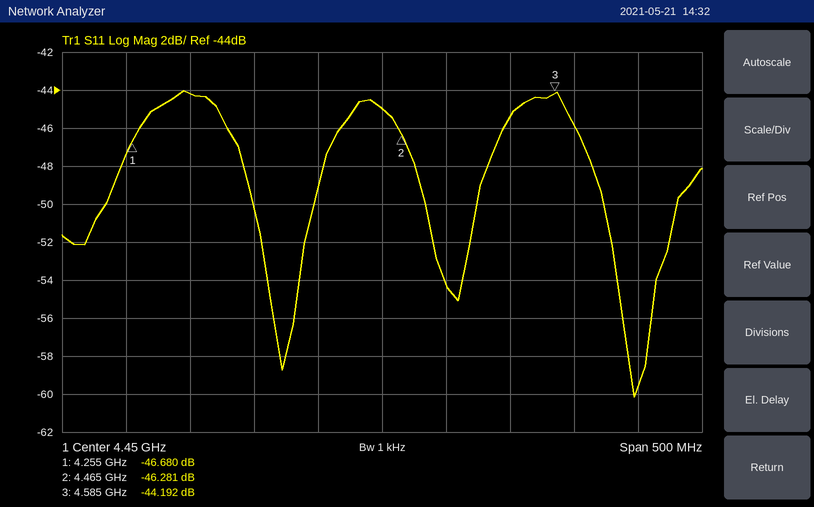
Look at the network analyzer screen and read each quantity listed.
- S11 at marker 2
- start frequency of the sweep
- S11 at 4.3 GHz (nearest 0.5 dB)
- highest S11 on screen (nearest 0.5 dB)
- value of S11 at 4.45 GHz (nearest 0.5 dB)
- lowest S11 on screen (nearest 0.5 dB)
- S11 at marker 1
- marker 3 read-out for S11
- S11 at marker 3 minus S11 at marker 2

-46.281 dB
4.2 GHz
-44.0 dB
-44.0 dB
-45.0 dB
-60.0 dB
-46.680 dB
-44.192 dB
2.089 dB
